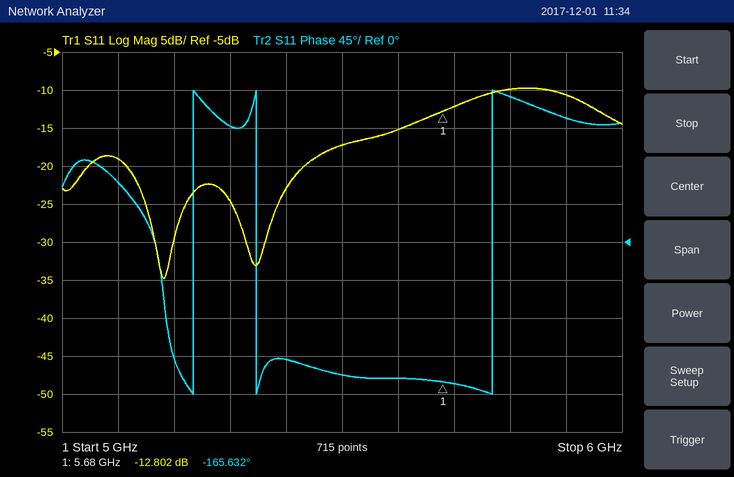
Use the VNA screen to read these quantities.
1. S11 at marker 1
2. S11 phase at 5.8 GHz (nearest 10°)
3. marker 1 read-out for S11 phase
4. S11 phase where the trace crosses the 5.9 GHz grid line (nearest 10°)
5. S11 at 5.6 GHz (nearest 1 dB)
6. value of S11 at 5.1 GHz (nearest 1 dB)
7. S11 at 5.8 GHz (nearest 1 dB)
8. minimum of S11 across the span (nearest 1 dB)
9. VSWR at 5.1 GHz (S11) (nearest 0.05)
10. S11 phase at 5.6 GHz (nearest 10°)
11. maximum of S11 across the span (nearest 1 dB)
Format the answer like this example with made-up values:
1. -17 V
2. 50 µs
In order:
1. -12.802 dB
2. 170°
3. -165.632°
4. 150°
5. -15 dB
6. -19 dB
7. -10 dB
8. -35 dB
9. 1.25
10. -160°
11. -10 dB
